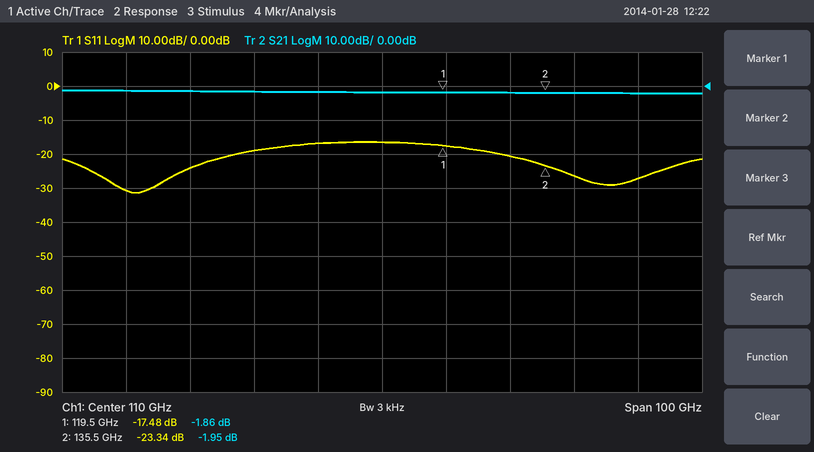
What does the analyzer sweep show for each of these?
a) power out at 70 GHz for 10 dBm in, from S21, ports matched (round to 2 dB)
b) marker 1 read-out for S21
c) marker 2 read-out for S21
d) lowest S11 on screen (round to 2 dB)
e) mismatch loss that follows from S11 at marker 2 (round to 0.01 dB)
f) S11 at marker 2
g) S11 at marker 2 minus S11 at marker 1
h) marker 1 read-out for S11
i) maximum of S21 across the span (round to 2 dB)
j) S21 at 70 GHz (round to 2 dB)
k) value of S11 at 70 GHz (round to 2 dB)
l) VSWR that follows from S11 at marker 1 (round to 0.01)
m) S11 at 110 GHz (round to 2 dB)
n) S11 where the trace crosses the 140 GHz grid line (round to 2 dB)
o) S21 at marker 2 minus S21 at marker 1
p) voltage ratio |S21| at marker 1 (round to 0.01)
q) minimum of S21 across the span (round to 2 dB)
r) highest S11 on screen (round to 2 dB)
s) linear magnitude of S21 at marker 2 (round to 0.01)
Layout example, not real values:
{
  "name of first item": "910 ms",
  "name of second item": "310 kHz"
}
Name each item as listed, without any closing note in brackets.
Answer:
{
  "power out at 70 GHz for 10 dBm in, from S21, ports matched": "8 dBm",
  "marker 1 read-out for S21": "-1.86 dB",
  "marker 2 read-out for S21": "-1.95 dB",
  "lowest S11 on screen": "-32 dB",
  "mismatch loss that follows from S11 at marker 2": "0.02 dB",
  "S11 at marker 2": "-23.34 dB",
  "S11 at marker 2 minus S11 at marker 1": "-5.86 dB",
  "marker 1 read-out for S11": "-17.48 dB",
  "maximum of S21 across the span": "-2 dB",
  "S21 at 70 GHz": "-2 dB",
  "value of S11 at 70 GHz": "-30 dB",
  "VSWR that follows from S11 at marker 1": "1.31",
  "S11 at 110 GHz": "-16 dB",
  "S11 where the trace crosses the 140 GHz grid line": "-26 dB",
  "S21 at marker 2 minus S21 at marker 1": "-0.09 dB",
  "voltage ratio |S21| at marker 1": "0.81",
  "minimum of S21 across the span": "-2 dB",
  "highest S11 on screen": "-16 dB",
  "linear magnitude of S21 at marker 2": "0.80"
}
